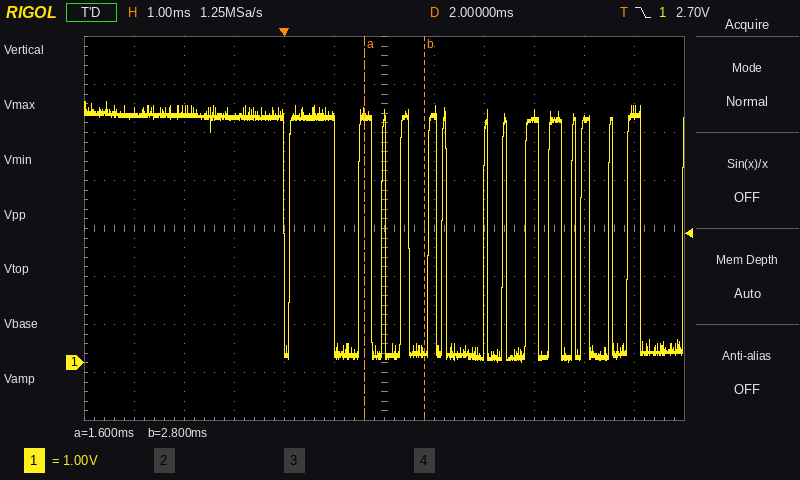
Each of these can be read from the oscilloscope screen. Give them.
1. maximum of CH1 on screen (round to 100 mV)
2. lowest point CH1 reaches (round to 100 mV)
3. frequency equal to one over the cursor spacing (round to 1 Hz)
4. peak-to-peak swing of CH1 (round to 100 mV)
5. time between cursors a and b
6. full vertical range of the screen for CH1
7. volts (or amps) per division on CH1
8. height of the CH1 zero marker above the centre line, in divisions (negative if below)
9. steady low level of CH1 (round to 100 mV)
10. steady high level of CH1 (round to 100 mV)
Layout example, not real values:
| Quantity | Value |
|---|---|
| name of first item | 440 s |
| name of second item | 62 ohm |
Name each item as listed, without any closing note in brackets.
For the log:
| Quantity | Value |
|---|---|
| maximum of CH1 on screen | 5.4 V |
| lowest point CH1 reaches | 0.0 V |
| frequency equal to one over the cursor spacing | 833 Hz |
| peak-to-peak swing of CH1 | 5.4 V |
| time between cursors a and b | 1.2 ms |
| full vertical range of the screen for CH1 | 8 V |
| volts (or amps) per division on CH1 | 1 V |
| height of the CH1 zero marker above the centre line, in divisions | -2.8 div |
| steady low level of CH1 | 200 mV |
| steady high level of CH1 | 5.2 V |
